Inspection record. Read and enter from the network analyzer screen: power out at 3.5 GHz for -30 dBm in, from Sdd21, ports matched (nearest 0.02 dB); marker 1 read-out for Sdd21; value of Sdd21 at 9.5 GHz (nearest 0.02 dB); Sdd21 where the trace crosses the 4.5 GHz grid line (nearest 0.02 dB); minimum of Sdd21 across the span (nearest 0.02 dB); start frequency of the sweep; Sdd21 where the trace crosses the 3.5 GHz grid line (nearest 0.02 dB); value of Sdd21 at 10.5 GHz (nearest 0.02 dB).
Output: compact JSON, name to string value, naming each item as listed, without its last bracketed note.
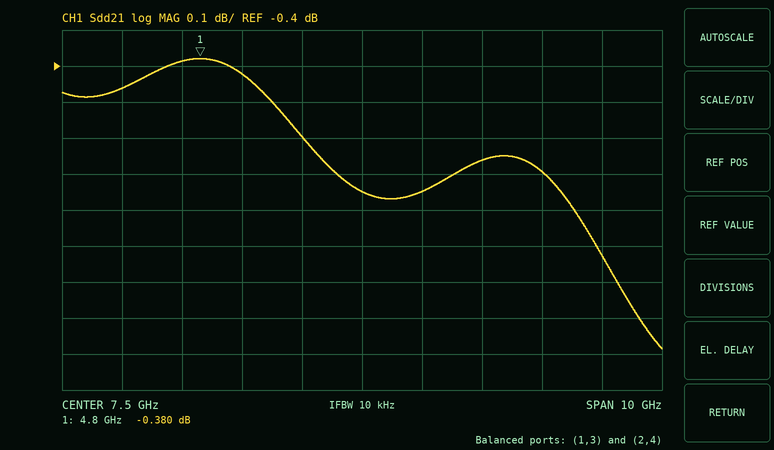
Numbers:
{"power out at 3.5 GHz for -30 dBm in, from Sdd21, ports matched": "-30.46 dBm", "marker 1 read-out for Sdd21": "-0.380 dB", "value of Sdd21 at 9.5 GHz": "-0.66 dB", "Sdd21 where the trace crosses the 4.5 GHz grid line": "-0.38 dB", "minimum of Sdd21 across the span": "-1.18 dB", "start frequency of the sweep": "2.5 GHz", "Sdd21 where the trace crosses the 3.5 GHz grid line": "-0.46 dB", "value of Sdd21 at 10.5 GHz": "-0.70 dB"}
